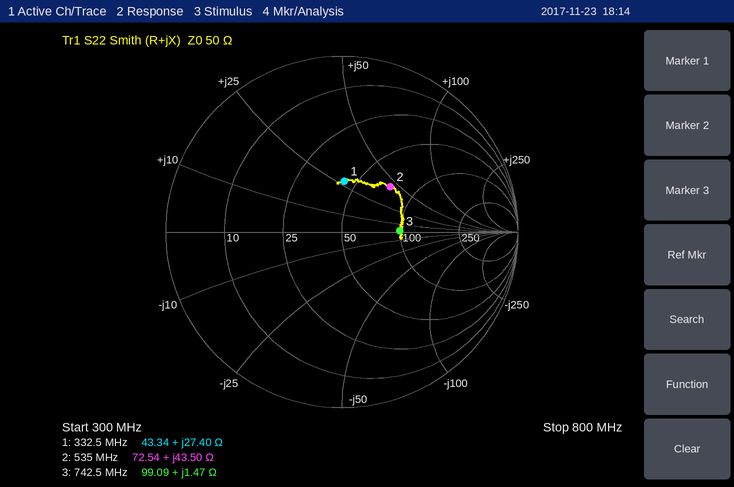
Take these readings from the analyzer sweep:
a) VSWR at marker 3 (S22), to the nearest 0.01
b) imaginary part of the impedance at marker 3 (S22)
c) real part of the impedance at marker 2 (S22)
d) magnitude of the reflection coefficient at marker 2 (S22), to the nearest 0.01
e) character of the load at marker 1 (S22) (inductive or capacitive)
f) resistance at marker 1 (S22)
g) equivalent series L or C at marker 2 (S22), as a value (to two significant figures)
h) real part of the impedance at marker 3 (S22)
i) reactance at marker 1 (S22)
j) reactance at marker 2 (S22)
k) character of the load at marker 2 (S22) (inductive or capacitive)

1.98
+1.47 Ω
72.54 Ω
0.38
inductive
43.34 Ω
13 nH
99.09 Ω
+27.40 Ω
+43.50 Ω
inductive
